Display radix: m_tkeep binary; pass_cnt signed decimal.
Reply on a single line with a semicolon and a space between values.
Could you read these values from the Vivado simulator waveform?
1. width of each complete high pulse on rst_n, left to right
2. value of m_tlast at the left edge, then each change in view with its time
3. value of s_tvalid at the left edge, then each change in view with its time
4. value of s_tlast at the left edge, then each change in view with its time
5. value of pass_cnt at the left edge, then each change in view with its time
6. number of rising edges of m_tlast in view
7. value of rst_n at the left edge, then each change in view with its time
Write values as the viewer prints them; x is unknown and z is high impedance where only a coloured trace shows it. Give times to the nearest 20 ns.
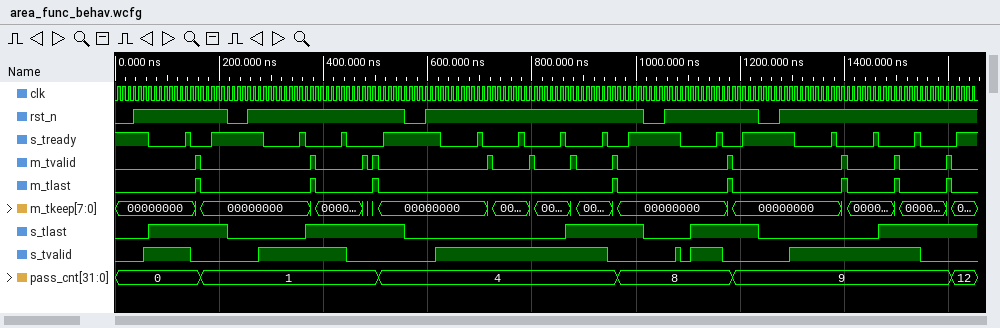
180 ns, 300 ns, 420 ns, 180 ns; 0, 1 at 160 ns, 0 at 160 ns, 1 at 380 ns, 0 at 380 ns, 1 at 500 ns, 0 at 500 ns, 1 at 960 ns, 0 at 960 ns, 1 at 1180 ns, 0 at 1180 ns, 1 at 1400 ns, 0 at 1400 ns, 1 at 1500 ns, 0 at 1500 ns, 1 at 1600 ns, 0 at 1600 ns; 0, 1 at 60 ns, 0 at 140 ns, 1 at 280 ns, 0 at 440 ns, 1 at 620 ns, 0 at 940 ns, 1 at 1080 ns, 0 at 1080 ns, 1 at 1100 ns, 0 at 1160 ns, 1 at 1300 ns, 0 at 1540 ns; 0, 1 at 60 ns, 0 at 220 ns, 1 at 360 ns, 0 at 560 ns, 1 at 860 ns, 0 at 1020 ns, 1 at 1100 ns, 0 at 1240 ns, 1 at 1460 ns; 0, 1 at 160 ns, 4 at 500 ns, 8 at 960 ns, 9 at 1180 ns, 12 at 1600 ns; 8; 0, 1 at 40 ns, 0 at 220 ns, 1 at 260 ns, 0 at 560 ns, 1 at 600 ns, 0 at 1020 ns, 1 at 1060 ns, 0 at 1240 ns, 1 at 1280 ns
